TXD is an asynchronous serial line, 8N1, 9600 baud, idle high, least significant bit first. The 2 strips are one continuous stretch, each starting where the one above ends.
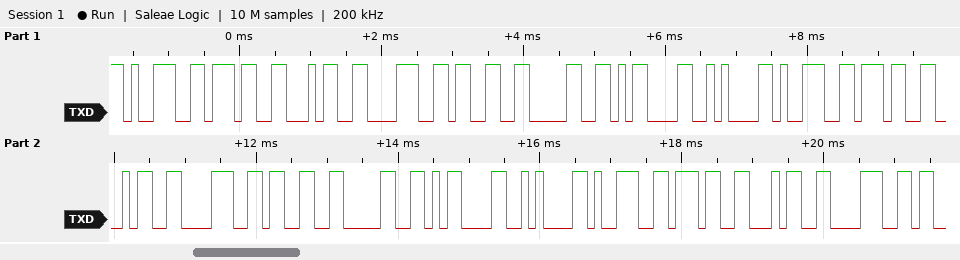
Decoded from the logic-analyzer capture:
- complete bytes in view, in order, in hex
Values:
0x39 0x37 0x34 0x38 0x33 0x30 0x0D 0x0A 0x39 0x37 0x34 0x38 0x33 0x30 0x0D 0x0A 0x39 0x37 0x34 0x38
